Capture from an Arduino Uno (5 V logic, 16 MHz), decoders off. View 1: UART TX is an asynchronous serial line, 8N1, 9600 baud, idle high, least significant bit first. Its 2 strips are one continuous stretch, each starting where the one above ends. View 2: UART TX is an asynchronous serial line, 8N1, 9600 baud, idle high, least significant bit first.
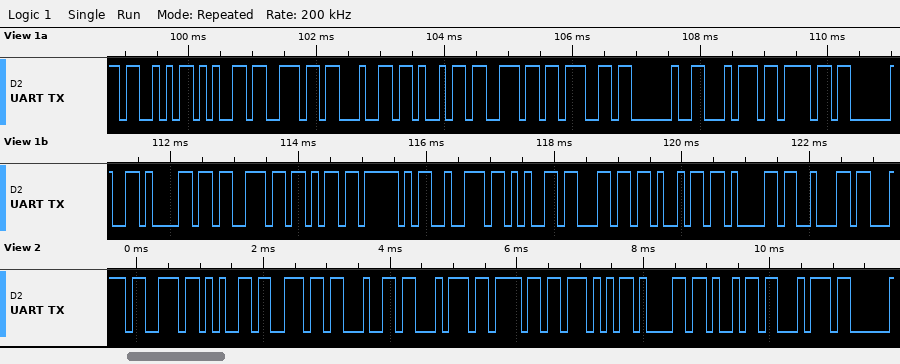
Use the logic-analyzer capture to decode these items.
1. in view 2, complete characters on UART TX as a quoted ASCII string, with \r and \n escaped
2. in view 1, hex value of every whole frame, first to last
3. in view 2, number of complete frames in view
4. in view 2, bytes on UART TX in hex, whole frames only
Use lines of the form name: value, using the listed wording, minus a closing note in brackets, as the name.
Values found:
in view 2, complete characters on UART TX as a quoted ASCII string, with \r and \n escaped: "sendtoWait"
in view 1, hex value of every whole frame, first to last: 0x53 0x65 0x6E 0x64 0x69 0x6E 0x67 0x20 0x74 0x6F 0x20 0x61 0x73 0x6B 0x5F 0x72 0x65 0x6C 0x69 0x61 0x62
in view 2, number of complete frames in view: 10
in view 2, bytes on UART TX in hex, whole frames only: 73 65 6E 64 74 6F 57 61 69 74
